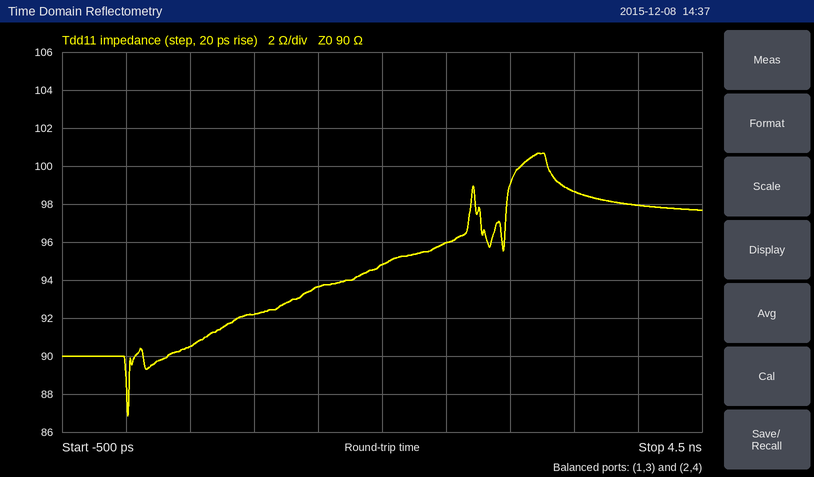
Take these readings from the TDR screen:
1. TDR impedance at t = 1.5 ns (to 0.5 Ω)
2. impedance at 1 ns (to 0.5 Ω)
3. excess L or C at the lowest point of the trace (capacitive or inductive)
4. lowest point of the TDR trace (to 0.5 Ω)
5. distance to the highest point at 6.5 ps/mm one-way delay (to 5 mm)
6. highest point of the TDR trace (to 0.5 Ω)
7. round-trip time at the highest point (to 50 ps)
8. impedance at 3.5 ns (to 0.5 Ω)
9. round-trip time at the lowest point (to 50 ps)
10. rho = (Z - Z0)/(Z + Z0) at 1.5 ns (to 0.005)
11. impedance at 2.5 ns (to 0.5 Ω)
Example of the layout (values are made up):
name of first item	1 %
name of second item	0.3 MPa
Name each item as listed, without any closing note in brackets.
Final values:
TDR impedance at t = 1.5 ns	93.5 Ω
impedance at 1 ns	92.0 Ω
excess L or C at the lowest point of the trace	capacitive
lowest point of the TDR trace	87.0 Ω
distance to the highest point at 6.5 ps/mm one-way delay	250 mm
highest point of the TDR trace	100.5 Ω
round-trip time at the highest point	3.25 ns
impedance at 3.5 ns	98.5 Ω
round-trip time at the lowest point	0 ps
rho = (Z - Z0)/(Z + Z0) at 1.5 ns	+0.020
impedance at 2.5 ns	96.0 Ω
